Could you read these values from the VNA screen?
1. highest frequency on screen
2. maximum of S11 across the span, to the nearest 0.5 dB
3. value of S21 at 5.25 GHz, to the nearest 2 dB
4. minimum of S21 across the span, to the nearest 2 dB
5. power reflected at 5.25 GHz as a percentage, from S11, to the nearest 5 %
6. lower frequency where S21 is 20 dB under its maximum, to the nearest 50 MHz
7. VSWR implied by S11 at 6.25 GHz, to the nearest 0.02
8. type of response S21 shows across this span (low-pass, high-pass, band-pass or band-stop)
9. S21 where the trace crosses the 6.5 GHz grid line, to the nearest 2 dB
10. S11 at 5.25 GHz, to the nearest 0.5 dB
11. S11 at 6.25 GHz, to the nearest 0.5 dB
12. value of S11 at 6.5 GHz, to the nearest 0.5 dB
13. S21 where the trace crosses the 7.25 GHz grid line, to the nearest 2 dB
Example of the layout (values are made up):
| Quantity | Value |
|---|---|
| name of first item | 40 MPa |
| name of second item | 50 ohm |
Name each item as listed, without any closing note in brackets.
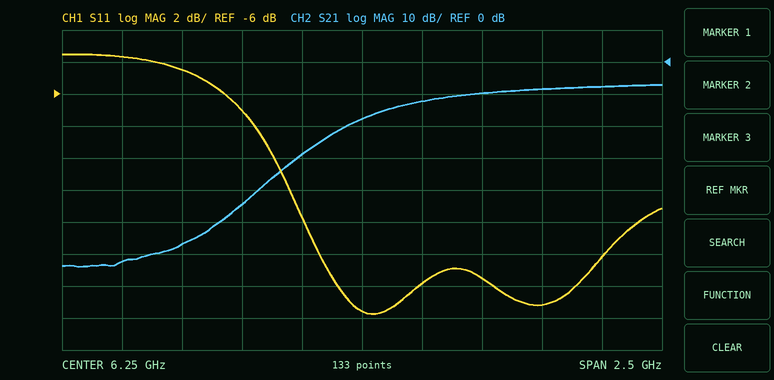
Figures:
| Quantity | Value |
|---|---|
| highest frequency on screen | 7.5 GHz |
| maximum of S11 across the span, to the nearest 0.5 dB | -3.5 dB |
| value of S21 at 5.25 GHz, to the nearest 2 dB | -62 dB |
| minimum of S21 across the span, to the nearest 2 dB | -64 dB |
| power reflected at 5.25 GHz as a percentage, from S11, to the nearest 5 % | 45 % |
| lower frequency where S21 is 20 dB under its maximum, to the nearest 50 MHz | 6.05 GHz |
| VSWR implied by S11 at 6.25 GHz, to the nearest 0.02 | 1.24 |
| type of response S21 shows across this span | high-pass |
| S21 where the trace crosses the 6.5 GHz grid line, to the nearest 2 dB | -12 dB |
| S11 at 5.25 GHz, to the nearest 0.5 dB | -3.5 dB |
| S11 at 6.25 GHz, to the nearest 0.5 dB | -19.5 dB |
| value of S11 at 6.5 GHz, to the nearest 0.5 dB | -18.0 dB |
| S21 where the trace crosses the 7.25 GHz grid line, to the nearest 2 dB | -8 dB |
